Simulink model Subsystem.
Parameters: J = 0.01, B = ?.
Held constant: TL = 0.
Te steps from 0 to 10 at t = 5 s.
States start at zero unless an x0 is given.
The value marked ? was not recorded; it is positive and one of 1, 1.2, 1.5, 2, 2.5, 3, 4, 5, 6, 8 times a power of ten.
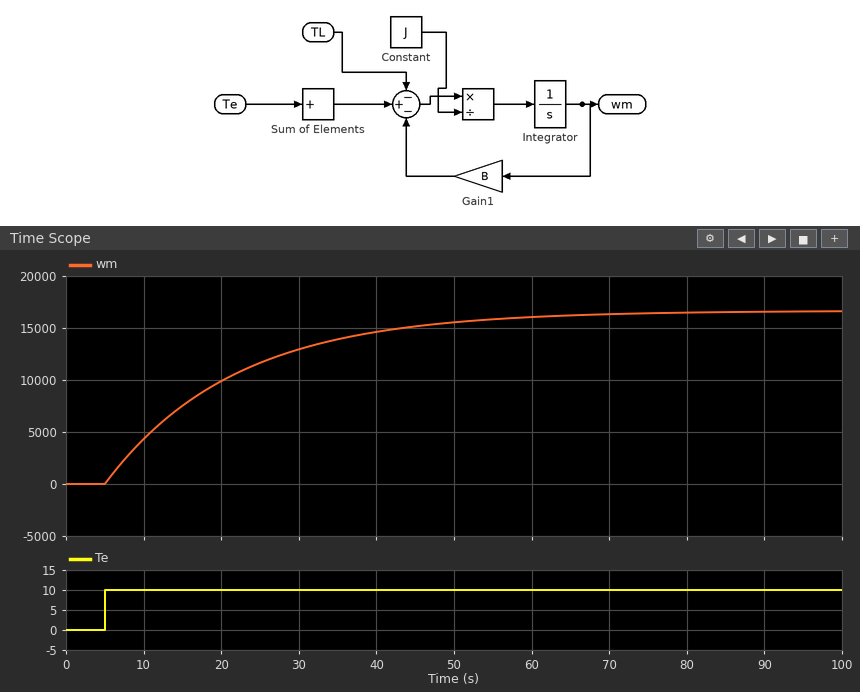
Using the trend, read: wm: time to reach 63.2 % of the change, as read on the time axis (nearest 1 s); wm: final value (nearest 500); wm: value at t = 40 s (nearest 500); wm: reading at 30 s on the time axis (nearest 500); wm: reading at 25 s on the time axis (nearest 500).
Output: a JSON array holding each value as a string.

["22 s", "16500", "14500", "13000", "11500"]
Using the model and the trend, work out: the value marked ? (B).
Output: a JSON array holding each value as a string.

["0.0006"]
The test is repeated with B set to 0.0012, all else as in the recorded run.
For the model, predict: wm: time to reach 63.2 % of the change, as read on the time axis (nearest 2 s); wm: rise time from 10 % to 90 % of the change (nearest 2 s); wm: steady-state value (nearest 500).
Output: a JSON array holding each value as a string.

["14 s", "18 s", "8500"]
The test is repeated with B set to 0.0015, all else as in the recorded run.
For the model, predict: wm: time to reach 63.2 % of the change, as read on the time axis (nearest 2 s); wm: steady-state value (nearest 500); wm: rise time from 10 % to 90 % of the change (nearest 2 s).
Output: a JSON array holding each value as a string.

["12 s", "6500", "14 s"]
